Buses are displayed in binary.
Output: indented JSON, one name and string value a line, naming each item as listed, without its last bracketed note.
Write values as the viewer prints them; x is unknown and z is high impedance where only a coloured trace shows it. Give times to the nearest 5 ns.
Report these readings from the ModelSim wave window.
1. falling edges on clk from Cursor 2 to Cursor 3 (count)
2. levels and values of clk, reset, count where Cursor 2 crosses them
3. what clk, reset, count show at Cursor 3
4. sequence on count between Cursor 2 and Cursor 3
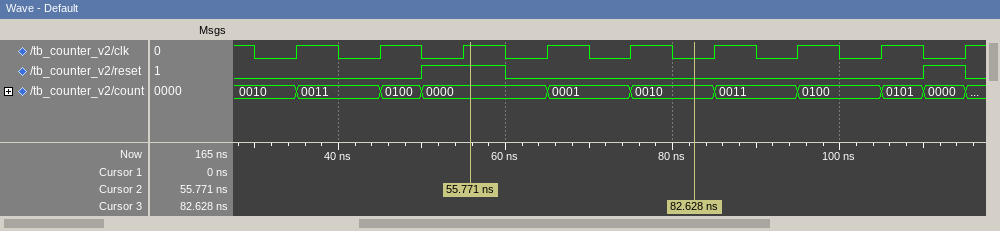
{
  "falling edges on clk from Cursor 2 to Cursor 3": "3",
  "levels and values of clk, reset, count where Cursor 2 crosses them": "clk=1, reset=1, count=0000",
  "what clk, reset, count show at Cursor 3": "clk=0, reset=0, count=0010",
  "sequence on count between Cursor 2 and Cursor 3": "0000, 0001, 0010"
}
